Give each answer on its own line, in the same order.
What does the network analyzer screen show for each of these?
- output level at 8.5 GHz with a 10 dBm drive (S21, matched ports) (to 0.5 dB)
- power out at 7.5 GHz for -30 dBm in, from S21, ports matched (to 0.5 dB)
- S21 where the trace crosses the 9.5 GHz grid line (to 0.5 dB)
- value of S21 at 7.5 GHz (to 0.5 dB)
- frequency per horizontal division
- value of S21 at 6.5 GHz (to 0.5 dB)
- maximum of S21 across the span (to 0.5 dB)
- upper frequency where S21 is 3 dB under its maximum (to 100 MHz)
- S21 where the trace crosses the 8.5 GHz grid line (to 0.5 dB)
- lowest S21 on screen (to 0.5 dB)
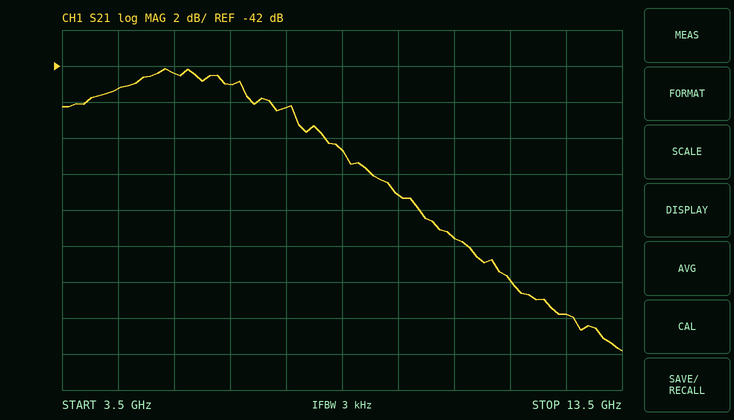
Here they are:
-36.5 dBm
-74.5 dBm
-49.0 dB
-44.5 dB
1 GHz
-43.0 dB
-42.0 dB
7.7 GHz
-46.5 dB
-58.0 dB
